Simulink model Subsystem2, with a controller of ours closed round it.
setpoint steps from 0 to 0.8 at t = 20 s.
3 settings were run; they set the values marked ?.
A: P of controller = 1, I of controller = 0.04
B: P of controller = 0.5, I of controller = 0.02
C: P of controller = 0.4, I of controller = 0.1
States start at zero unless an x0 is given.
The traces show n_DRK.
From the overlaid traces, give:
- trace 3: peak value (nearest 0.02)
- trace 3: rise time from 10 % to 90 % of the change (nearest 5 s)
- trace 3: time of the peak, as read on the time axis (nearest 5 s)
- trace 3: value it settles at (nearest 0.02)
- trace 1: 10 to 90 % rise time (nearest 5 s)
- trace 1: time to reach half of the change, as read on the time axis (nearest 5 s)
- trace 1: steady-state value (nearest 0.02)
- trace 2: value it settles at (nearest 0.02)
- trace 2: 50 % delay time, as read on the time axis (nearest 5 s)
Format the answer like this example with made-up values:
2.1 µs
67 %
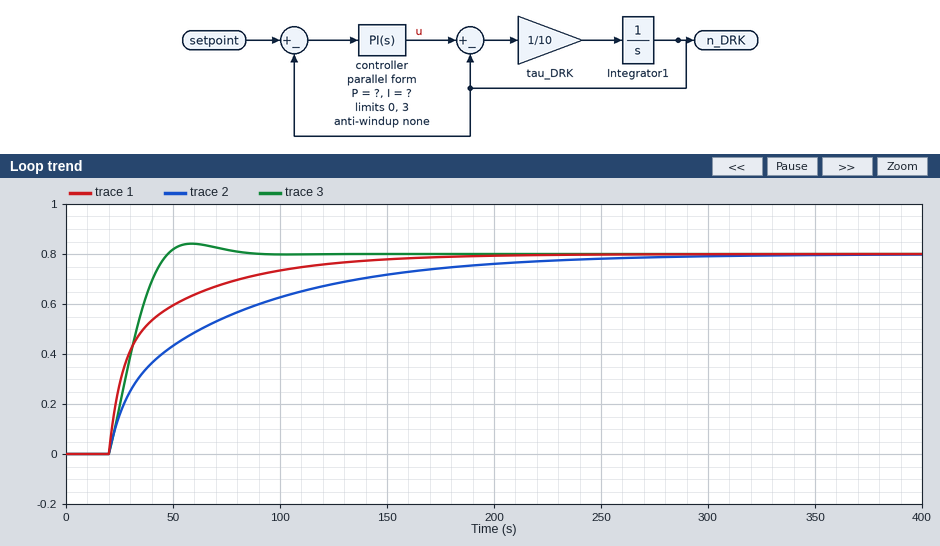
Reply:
0.84
20 s
60 s
0.80
70 s
30 s
0.80
0.80
45 s
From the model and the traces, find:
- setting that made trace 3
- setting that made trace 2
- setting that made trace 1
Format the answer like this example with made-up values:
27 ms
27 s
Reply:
C
B
A
